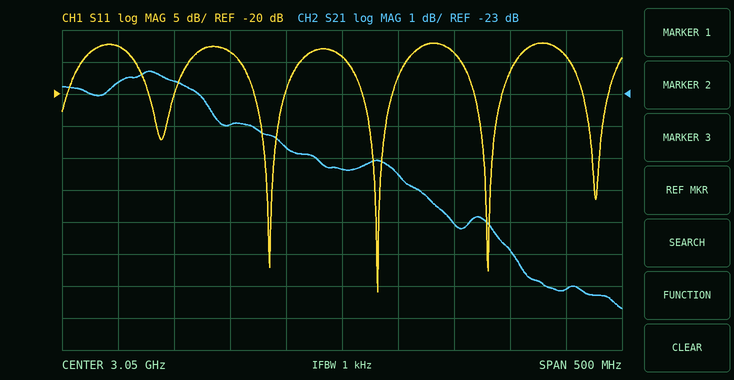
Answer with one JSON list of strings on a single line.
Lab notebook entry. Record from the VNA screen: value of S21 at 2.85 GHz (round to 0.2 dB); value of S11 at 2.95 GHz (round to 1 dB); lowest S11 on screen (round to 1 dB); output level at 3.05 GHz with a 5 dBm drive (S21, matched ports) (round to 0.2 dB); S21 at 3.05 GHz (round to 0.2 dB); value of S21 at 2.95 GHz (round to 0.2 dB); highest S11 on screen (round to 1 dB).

["-22.6 dB", "-13 dB", "-51 dB", "-20.4 dBm", "-25.4 dB", "-24.0 dB", "-12 dB"]
